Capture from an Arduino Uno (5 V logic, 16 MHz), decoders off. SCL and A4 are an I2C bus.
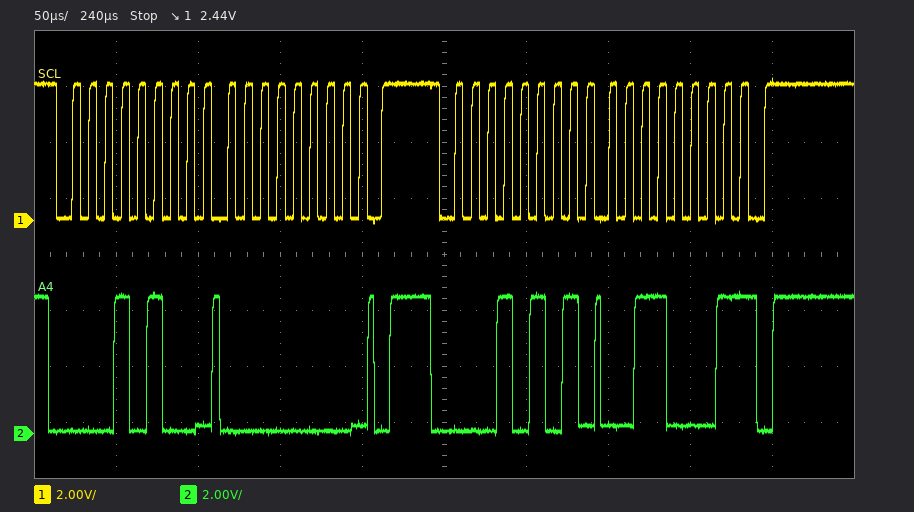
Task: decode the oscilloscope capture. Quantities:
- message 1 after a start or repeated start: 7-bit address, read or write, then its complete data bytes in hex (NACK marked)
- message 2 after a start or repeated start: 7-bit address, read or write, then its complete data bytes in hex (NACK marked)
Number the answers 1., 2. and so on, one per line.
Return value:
1. 0x0A write: 00
2. 0x0A read: 31 NACK
